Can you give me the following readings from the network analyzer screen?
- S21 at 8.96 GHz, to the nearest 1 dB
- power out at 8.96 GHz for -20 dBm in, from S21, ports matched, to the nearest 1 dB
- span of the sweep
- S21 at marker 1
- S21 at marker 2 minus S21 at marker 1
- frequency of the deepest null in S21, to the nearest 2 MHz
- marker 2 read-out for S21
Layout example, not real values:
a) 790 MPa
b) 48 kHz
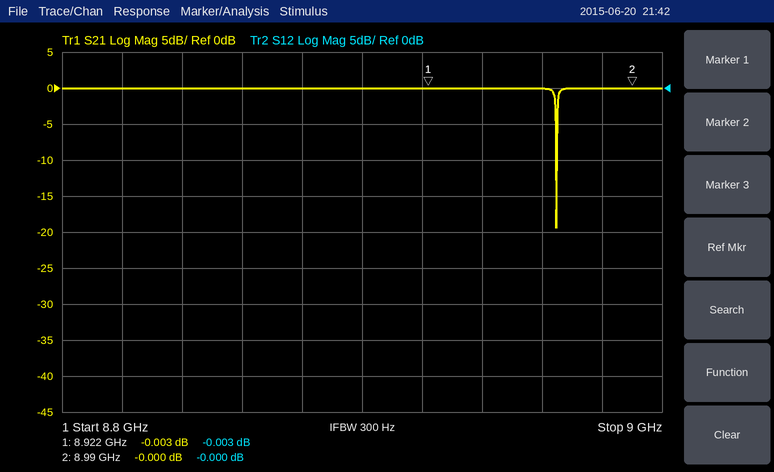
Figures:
a) 0 dB
b) -20 dBm
c) 200 MHz
d) -0.003 dB
e) 0.003 dB
f) 8.964 GHz
g) -0.000 dB
